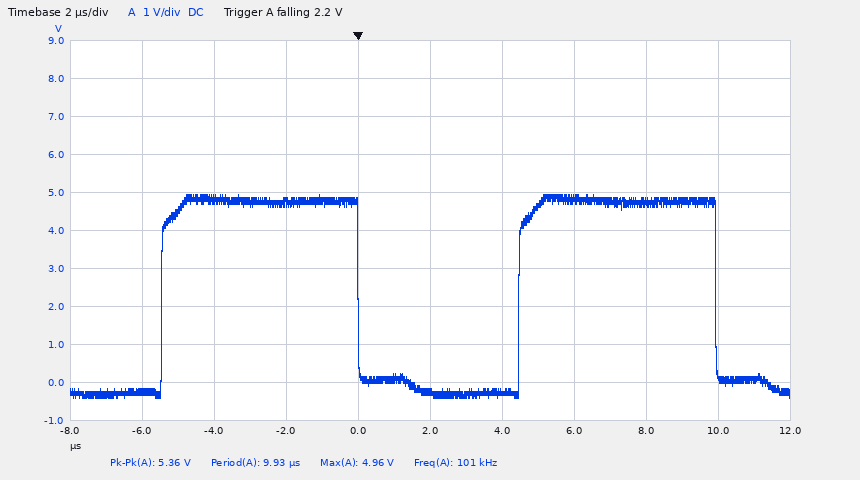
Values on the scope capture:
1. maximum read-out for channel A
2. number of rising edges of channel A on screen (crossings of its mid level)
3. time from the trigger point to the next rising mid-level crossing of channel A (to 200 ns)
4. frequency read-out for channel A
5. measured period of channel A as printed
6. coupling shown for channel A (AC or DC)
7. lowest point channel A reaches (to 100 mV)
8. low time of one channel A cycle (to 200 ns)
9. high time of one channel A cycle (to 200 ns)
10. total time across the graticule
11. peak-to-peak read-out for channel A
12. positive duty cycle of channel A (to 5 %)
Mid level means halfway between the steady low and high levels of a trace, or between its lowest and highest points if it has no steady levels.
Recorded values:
4.96 V
2
4.4 µs
101 kHz
9.93 µs
DC
-400 mV
4.4 µs
5.4 µs
20 µs
5.36 V
55 %
